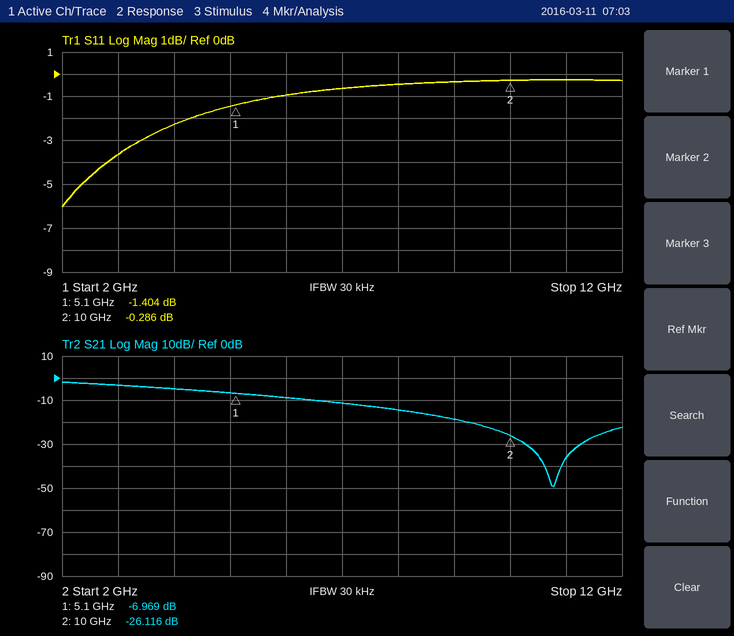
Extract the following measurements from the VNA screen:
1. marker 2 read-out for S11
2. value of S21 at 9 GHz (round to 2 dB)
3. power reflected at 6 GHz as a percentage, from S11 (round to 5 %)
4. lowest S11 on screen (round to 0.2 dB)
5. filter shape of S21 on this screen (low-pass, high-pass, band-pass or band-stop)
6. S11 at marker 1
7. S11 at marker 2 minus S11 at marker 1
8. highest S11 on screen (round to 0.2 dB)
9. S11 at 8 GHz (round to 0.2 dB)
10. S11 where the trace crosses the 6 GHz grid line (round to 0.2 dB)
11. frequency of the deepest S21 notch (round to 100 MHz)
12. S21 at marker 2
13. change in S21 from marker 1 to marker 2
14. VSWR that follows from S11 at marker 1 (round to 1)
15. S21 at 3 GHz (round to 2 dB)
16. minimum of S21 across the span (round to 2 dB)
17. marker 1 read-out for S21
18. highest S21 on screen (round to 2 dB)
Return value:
-0.286 dB
-18 dB
80 %
-6.0 dB
low-pass
-1.404 dB
1.118 dB
-0.2 dB
-0.4 dB
-1.0 dB
10.8 GHz
-26.116 dB
-19.147 dB
12
-4 dB
-50 dB
-6.969 dB
-2 dB
